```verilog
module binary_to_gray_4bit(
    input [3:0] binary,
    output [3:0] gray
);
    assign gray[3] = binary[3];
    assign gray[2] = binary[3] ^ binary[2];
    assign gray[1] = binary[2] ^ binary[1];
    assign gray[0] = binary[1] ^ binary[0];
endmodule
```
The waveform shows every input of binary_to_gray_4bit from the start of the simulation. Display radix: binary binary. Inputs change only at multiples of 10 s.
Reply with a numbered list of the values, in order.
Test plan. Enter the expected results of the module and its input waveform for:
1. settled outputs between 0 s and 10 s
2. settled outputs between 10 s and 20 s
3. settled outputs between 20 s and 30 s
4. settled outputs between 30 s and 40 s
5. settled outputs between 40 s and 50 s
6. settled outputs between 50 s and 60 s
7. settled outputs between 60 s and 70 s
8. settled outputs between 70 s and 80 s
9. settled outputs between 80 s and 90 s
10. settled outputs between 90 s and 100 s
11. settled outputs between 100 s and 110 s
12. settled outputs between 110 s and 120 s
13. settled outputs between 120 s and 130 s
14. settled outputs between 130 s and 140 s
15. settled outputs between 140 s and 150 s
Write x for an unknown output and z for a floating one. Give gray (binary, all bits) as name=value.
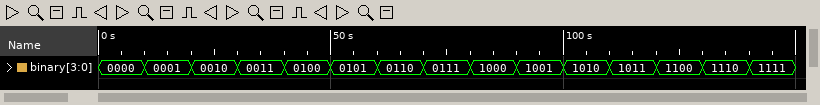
1. gray=0000
2. gray=0001
3. gray=0011
4. gray=0010
5. gray=0110
6. gray=0111
7. gray=0101
8. gray=0100
9. gray=1100
10. gray=1101
11. gray=1111
12. gray=1110
13. gray=1010
14. gray=1001
15. gray=1000
